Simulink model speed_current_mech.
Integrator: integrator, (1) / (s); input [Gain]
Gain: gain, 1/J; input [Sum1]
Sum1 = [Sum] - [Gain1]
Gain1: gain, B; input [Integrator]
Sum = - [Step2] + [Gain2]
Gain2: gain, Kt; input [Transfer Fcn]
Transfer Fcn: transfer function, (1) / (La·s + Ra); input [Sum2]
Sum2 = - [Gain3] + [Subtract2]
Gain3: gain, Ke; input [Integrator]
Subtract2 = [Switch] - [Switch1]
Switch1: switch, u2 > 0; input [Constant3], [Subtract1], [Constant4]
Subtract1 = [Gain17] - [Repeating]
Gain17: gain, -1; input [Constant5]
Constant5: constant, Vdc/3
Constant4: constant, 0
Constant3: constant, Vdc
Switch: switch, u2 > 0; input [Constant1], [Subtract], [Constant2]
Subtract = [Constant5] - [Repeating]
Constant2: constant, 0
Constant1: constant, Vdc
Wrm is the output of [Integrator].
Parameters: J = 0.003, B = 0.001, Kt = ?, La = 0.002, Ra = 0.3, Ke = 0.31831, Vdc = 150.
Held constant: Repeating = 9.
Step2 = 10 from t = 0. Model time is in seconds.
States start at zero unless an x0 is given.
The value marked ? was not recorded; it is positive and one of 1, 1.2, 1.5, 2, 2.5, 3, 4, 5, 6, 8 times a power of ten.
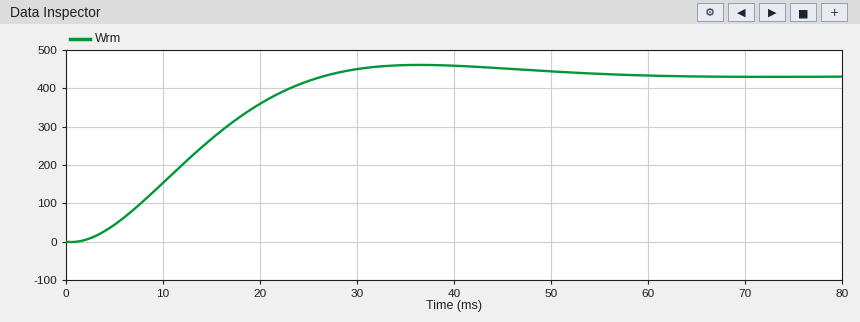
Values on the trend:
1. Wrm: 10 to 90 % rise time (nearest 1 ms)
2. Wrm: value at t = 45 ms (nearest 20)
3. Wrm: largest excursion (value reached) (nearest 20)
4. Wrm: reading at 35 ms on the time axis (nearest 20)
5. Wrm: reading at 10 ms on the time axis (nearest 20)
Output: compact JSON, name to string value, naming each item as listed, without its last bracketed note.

{"Wrm: 10 to 90 % rise time": "17 ms", "Wrm: value at t = 45 ms": "460", "Wrm: largest excursion (value reached)": "460", "Wrm: reading at 35 ms on the time axis": "460", "Wrm: reading at 10 ms on the time axis": "160"}
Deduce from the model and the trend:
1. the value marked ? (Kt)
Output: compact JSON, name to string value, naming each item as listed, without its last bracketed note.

{"the value marked ?": "0.25"}
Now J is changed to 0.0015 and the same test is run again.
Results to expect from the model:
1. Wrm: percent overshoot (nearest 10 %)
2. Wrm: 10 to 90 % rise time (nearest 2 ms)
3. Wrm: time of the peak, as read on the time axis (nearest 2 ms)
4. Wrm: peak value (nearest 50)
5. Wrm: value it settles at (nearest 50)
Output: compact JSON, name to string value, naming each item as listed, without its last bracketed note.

{"Wrm: percent overshoot": "20 %", "Wrm: 10 to 90 % rise time": "10 ms", "Wrm: time of the peak, as read on the time axis": "22 ms", "Wrm: peak value": "500", "Wrm: value it settles at": "450"}
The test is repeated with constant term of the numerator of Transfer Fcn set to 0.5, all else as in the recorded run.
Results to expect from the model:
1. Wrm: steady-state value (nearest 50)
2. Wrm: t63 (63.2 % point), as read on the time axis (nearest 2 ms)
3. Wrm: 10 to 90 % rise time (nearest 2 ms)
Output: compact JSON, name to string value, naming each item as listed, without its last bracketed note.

{"Wrm: steady-state value": "400", "Wrm: t63 (63.2 % point), as read on the time axis": "26 ms", "Wrm: 10 to 90 % rise time": "36 ms"}
